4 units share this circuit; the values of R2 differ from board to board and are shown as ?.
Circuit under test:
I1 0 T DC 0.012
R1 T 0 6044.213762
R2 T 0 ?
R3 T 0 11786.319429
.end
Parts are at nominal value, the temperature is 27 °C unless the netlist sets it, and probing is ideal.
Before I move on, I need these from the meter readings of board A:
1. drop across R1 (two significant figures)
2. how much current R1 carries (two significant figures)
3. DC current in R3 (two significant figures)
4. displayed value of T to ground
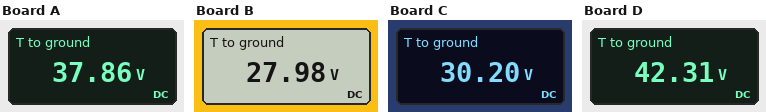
38 V
6.3 mA
3.2 mA
37.86 V
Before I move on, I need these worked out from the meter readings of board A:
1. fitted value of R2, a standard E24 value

15 kΩ
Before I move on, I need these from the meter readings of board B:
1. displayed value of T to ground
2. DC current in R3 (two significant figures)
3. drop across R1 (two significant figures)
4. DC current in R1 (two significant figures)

27.98 V
2.4 mA
28 V
4.6 mA
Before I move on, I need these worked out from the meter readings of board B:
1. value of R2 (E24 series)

5.6 kΩ
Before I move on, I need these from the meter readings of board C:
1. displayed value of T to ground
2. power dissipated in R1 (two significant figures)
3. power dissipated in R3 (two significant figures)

30.20 V
150 mW
77 mW
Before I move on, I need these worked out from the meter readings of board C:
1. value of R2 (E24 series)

6.8 kΩ
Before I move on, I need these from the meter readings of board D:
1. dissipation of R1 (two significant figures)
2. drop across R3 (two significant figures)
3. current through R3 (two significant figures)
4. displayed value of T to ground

300 mW
42 V
3.6 mA
42.31 V
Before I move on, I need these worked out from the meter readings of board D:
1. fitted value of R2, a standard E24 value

30 kΩ
